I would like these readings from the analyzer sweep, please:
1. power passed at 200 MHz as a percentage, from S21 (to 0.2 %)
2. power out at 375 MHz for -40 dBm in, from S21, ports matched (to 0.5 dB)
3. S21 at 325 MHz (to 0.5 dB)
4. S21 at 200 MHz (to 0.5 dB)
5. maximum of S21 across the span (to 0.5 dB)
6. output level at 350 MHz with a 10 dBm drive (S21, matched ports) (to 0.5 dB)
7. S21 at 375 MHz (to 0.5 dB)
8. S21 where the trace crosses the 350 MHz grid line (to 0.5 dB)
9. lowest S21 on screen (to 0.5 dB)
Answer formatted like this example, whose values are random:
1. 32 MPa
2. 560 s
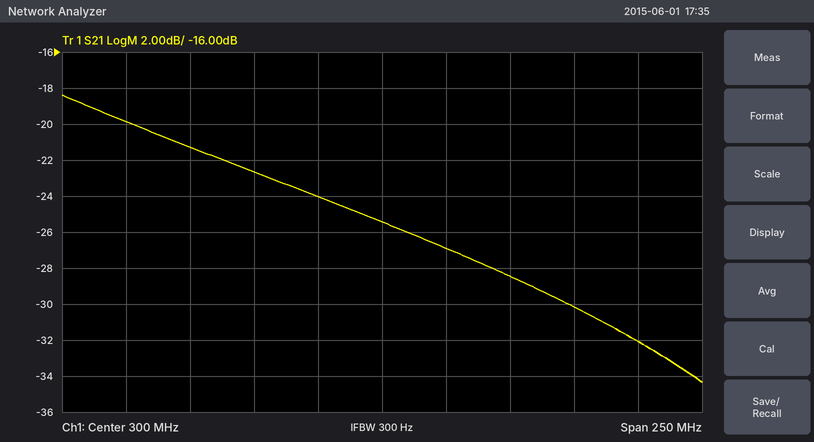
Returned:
1. 1.0 %
2. -70.0 dBm
3. -27.0 dB
4. -20.0 dB
5. -18.5 dB
6. -18.5 dBm
7. -30.0 dB
8. -28.5 dB
9. -34.5 dB
